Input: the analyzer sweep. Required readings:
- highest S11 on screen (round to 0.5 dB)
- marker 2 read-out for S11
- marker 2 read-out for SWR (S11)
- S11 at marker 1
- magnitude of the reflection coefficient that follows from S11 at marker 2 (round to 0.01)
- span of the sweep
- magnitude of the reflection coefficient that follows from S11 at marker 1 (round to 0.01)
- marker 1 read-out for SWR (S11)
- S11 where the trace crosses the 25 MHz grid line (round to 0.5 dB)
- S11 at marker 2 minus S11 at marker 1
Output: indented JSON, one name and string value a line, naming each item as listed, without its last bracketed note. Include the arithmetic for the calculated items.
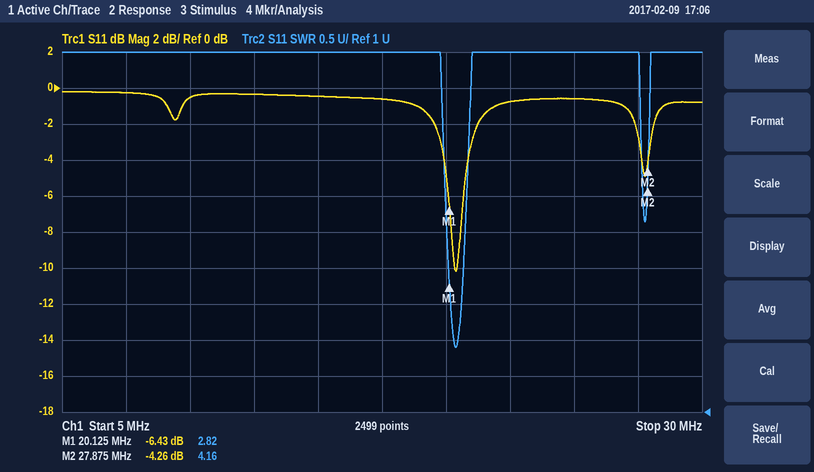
{
  "highest S11 on screen": "0.0 dB",
  "marker 2 read-out for S11": "-4.26 dB",
  "marker 2 read-out for SWR": "4.16",
  "S11 at marker 1": "-6.43 dB",
  "magnitude of the reflection coefficient that follows from S11 at marker 2": "10^(-4.26/20) ≈ 0.61",
  "span of the sweep": "25 MHz",
  "magnitude of the reflection coefficient that follows from S11 at marker 1": "10^(-6.43/20) ≈ 0.48",
  "marker 1 read-out for SWR": "2.82",
  "S11 where the trace crosses the 25 MHz grid line": "-0.5 dB",
  "S11 at marker 2 minus S11 at marker 1": "-4.26 − (-6.43) = 2.17 dB"
}
